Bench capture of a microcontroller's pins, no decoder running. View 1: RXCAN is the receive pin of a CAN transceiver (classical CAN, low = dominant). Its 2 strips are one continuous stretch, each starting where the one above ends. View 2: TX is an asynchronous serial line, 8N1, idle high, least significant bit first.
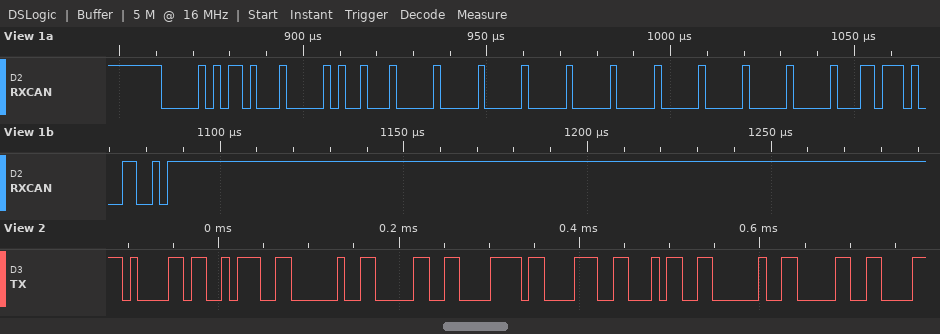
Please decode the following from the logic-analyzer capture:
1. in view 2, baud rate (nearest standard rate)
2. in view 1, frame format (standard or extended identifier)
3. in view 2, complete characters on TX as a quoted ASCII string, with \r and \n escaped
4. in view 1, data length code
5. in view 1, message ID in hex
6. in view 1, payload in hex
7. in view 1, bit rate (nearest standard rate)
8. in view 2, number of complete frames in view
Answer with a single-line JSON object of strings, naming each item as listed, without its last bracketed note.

{"in view 2, baud rate": "115200 baud", "in view 1, frame format": "standard", "in view 2, complete characters on TX as a quoted ASCII string, with \\r and \\n escaped": "\"a: 0x84 0\"", "in view 1, data length code": "8", "in view 1, message ID in hex": "0x02D", "in view 1, payload in hex": "12 20 00 00 00 00 00 00", "in view 1, bit rate": "500 kbit/s", "in view 2, number of complete frames in view": "9"}
